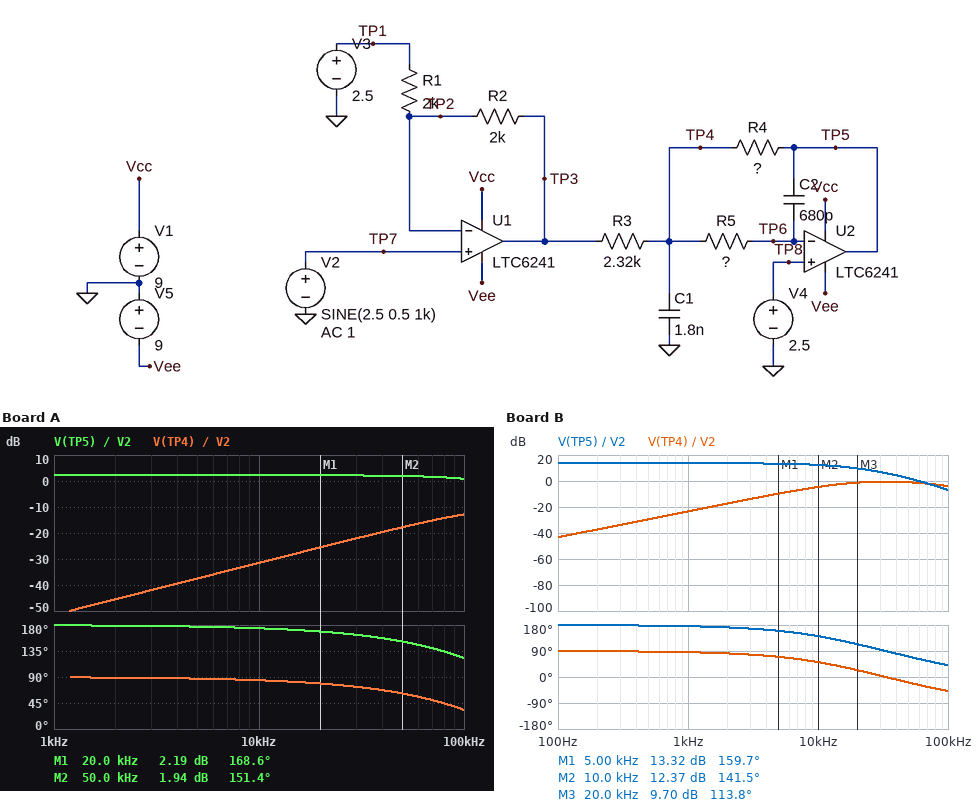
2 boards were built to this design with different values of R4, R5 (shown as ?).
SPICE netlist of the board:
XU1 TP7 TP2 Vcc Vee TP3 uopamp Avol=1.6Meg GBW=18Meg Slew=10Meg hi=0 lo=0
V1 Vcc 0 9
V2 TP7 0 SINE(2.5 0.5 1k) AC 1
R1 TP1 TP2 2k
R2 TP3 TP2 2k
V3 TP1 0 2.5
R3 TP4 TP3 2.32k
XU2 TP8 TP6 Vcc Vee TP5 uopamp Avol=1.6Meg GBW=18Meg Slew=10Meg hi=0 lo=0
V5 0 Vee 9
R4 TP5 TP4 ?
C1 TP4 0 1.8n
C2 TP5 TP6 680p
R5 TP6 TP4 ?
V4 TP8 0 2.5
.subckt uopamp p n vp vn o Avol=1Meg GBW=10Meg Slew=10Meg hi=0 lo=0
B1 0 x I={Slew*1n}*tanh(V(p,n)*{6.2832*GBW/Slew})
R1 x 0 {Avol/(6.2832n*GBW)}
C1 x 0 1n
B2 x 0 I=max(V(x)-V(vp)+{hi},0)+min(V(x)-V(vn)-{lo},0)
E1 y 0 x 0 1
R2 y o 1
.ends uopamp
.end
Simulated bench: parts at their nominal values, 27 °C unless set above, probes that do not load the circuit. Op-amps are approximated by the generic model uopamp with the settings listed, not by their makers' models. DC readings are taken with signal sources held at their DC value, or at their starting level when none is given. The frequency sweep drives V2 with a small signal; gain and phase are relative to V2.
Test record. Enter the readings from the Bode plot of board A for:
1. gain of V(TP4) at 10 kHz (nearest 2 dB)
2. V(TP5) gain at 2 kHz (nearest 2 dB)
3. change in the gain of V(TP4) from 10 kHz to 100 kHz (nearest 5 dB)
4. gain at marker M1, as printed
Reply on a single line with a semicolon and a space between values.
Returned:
-32 dB; 2 dB; 20 dB; 2.19 dB
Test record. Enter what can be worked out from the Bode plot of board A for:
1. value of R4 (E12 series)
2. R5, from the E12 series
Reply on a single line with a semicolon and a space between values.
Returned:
1.5 kΩ; 470 Ω
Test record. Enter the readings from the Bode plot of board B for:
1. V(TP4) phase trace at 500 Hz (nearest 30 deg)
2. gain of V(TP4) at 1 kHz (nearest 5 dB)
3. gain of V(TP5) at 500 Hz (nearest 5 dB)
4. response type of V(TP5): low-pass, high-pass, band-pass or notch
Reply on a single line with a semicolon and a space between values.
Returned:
90 deg; -25 dB; 15 dB; low-pass
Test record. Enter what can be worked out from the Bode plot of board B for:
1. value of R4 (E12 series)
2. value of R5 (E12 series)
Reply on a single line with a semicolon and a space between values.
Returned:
5.6 kΩ; 3.3 kΩ
